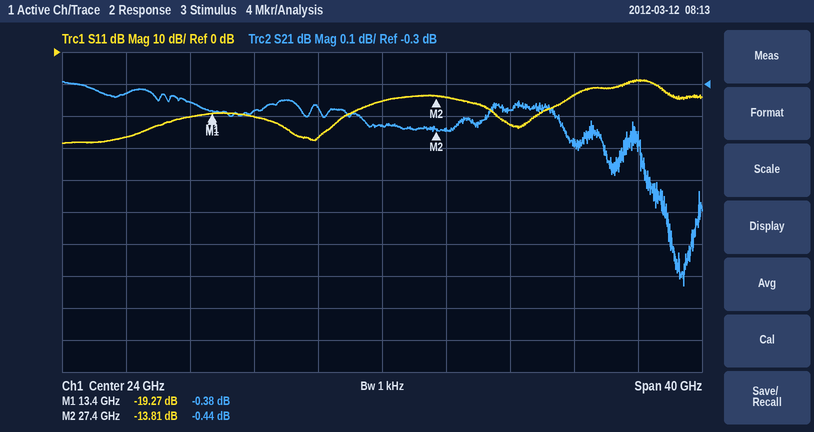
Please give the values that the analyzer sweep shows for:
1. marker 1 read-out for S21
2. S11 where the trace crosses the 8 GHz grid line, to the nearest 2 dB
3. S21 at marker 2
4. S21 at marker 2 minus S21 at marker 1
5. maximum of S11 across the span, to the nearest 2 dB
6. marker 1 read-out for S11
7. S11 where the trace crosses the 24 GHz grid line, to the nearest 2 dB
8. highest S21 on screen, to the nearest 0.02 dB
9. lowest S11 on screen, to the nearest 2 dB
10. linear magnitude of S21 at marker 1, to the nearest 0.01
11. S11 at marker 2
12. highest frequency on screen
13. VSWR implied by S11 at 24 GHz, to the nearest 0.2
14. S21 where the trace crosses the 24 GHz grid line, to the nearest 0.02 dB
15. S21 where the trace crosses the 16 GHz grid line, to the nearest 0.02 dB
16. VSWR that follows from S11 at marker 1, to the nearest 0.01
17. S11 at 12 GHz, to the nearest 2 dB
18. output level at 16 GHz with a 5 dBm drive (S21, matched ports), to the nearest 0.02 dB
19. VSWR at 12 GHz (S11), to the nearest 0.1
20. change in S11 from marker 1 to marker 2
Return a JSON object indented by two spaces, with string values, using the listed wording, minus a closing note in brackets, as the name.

{
  "marker 1 read-out for S21": "-0.38 dB",
  "S11 where the trace crosses the 8 GHz grid line, to the nearest 2 dB": "-26 dB",
  "S21 at marker 2": "-0.44 dB",
  "S21 at marker 2 minus S21 at marker 1": "-0.06 dB",
  "maximum of S11 across the span, to the nearest 2 dB": "-8 dB",
  "marker 1 read-out for S11": "-19.27 dB",
  "S11 where the trace crosses the 24 GHz grid line, to the nearest 2 dB": "-16 dB",
  "highest S21 on screen, to the nearest 0.02 dB": "-0.30 dB",
  "lowest S11 on screen, to the nearest 2 dB": "-28 dB",
  "linear magnitude of S21 at marker 1, to the nearest 0.01": "0.96",
  "S11 at marker 2": "-13.81 dB",
  "highest frequency on screen": "44 GHz",
  "VSWR implied by S11 at 24 GHz, to the nearest 0.2": "1.4",
  "S21 where the trace crosses the 24 GHz grid line, to the nearest 0.02 dB": "-0.44 dB",
  "S21 where the trace crosses the 16 GHz grid line, to the nearest 0.02 dB": "-0.38 dB",
  "VSWR that follows from S11 at marker 1, to the nearest 0.01": "1.24",
  "S11 at 12 GHz, to the nearest 2 dB": "-20 dB",
  "output level at 16 GHz with a 5 dBm drive (S21, matched ports), to the nearest 0.02 dB": "4.62 dBm",
  "VSWR at 12 GHz (S11), to the nearest 0.1": "1.2",
  "change in S11 from marker 1 to marker 2": "5.46 dB"
}
